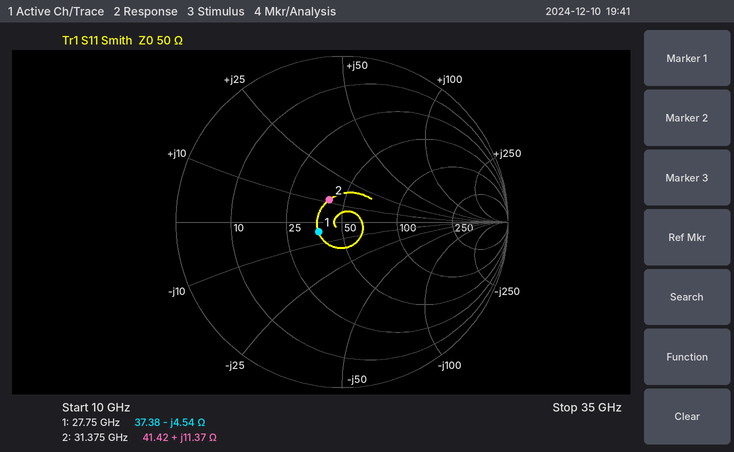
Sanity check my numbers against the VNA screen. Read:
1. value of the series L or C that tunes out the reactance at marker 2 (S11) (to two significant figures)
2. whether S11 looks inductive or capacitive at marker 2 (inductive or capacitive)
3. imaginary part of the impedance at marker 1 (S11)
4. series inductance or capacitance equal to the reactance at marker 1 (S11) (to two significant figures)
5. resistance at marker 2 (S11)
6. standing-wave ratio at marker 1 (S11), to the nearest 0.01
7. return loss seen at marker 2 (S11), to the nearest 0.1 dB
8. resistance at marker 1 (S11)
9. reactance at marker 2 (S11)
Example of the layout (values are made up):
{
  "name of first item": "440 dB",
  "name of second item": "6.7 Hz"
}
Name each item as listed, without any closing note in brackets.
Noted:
{
  "value of the series L or C that tunes out the reactance at marker 2 (S11)": "450 fF",
  "whether S11 looks inductive or capacitive at marker 2": "inductive",
  "imaginary part of the impedance at marker 1": "-4.54 Ω",
  "series inductance or capacitance equal to the reactance at marker 1 (S11)": "1.3 pF",
  "resistance at marker 2": "41.42 Ω",
  "standing-wave ratio at marker 1 (S11), to the nearest 0.01": "1.36",
  "return loss seen at marker 2 (S11), to the nearest 0.1 dB": "16.2 dB",
  "resistance at marker 1": "37.38 Ω",
  "reactance at marker 2": "+11.37 Ω"
}
